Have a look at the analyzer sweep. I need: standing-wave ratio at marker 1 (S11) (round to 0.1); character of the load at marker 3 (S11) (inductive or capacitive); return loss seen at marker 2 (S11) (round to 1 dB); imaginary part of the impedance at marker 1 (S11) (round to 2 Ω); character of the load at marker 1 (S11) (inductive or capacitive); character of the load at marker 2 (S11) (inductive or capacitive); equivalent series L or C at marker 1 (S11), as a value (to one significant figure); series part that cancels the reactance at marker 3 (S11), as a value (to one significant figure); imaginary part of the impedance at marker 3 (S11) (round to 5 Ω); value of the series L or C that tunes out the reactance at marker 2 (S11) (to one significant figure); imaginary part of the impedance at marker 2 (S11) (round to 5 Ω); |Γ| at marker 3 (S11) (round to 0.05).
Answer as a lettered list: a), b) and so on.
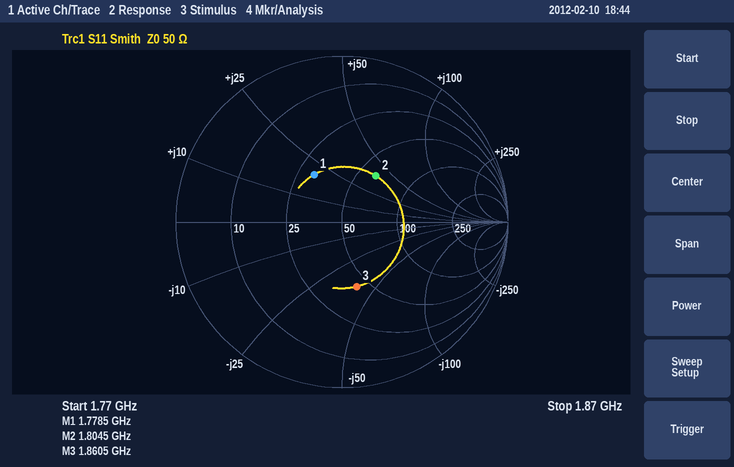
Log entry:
a) 2.0
b) capacitive
c) 9 dB
d) +20 Ω
e) inductive
f) inductive
g) 2 nH
h) 3 nH
i) -40 Ω
j) 2 pF
k) +40 Ω
l) 0.40
